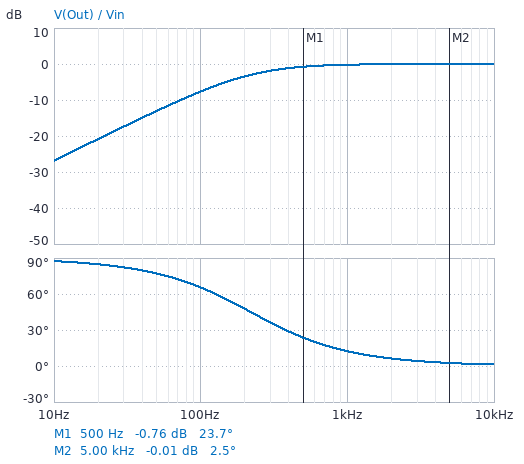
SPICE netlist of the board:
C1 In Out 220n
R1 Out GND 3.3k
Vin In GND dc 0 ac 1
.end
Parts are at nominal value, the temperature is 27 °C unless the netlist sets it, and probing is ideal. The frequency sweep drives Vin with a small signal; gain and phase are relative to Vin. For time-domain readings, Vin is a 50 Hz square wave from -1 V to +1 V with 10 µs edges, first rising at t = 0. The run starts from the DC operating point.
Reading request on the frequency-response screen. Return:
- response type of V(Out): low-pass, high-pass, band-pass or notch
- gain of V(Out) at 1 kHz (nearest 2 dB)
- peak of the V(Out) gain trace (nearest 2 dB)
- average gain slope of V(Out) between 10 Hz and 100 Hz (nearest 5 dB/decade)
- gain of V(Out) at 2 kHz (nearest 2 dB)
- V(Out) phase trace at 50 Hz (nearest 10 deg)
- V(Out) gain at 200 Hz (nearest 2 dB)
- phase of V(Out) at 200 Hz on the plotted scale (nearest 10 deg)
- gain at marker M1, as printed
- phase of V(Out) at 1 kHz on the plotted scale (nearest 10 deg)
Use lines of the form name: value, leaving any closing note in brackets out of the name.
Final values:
response type of V(Out): low-pass, high-pass, band-pass or notch: high-pass
gain of V(Out) at 1 kHz: 0 dB
peak of the V(Out) gain trace: 0 dB
average gain slope of V(Out) between 10 Hz and 100 Hz: 20 dB/decade
gain of V(Out) at 2 kHz: 0 dB
V(Out) phase trace at 50 Hz: 80 deg
V(Out) gain at 200 Hz: -4 dB
phase of V(Out) at 200 Hz on the plotted scale: 50 deg
gain at marker M1, as printed: -0.76 dB
phase of V(Out) at 1 kHz on the plotted scale: 10 deg
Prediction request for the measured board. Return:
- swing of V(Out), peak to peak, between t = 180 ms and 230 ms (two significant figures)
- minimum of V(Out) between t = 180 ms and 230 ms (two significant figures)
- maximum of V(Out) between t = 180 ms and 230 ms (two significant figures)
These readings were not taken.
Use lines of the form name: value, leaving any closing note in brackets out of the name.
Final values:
swing of V(Out), peak to peak, between t = 180 ms and 230 ms: 4.0 V
minimum of V(Out) between t = 180 ms and 230 ms: -2.0 V
maximum of V(Out) between t = 180 ms and 230 ms: 2.0 V
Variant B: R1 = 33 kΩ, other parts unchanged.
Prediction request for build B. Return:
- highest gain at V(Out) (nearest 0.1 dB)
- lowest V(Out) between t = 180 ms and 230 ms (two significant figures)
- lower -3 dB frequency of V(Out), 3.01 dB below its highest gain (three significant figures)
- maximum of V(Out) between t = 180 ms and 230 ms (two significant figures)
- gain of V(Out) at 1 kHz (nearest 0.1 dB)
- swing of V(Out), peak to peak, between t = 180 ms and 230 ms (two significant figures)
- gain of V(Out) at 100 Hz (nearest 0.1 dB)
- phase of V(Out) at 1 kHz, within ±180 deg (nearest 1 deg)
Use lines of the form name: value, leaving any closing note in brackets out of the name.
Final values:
highest gain at V(Out): 0 dB
lowest V(Out) between t = 180 ms and 230 ms: -1.6 V
lower -3 dB frequency of V(Out), 3.01 dB below its highest gain: 21.9 Hz
maximum of V(Out) between t = 180 ms and 230 ms: 1.6 V
gain of V(Out) at 1 kHz: 0 dB
swing of V(Out), peak to peak, between t = 180 ms and 230 ms: 3.2 V
gain of V(Out) at 100 Hz: -0.2 dB
phase of V(Out) at 1 kHz, within ±180 deg: 1 deg
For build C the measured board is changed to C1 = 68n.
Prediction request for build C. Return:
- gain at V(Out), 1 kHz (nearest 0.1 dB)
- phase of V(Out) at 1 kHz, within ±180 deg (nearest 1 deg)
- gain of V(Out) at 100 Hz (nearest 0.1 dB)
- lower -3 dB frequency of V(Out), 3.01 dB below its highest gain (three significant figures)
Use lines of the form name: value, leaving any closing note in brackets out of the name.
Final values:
gain at V(Out), 1 kHz: -1.8 dB
phase of V(Out) at 1 kHz, within ±180 deg: 35 deg
gain of V(Out) at 100 Hz: -17.1 dB
lower -3 dB frequency of V(Out), 3.01 dB below its highest gain: 709 Hz
